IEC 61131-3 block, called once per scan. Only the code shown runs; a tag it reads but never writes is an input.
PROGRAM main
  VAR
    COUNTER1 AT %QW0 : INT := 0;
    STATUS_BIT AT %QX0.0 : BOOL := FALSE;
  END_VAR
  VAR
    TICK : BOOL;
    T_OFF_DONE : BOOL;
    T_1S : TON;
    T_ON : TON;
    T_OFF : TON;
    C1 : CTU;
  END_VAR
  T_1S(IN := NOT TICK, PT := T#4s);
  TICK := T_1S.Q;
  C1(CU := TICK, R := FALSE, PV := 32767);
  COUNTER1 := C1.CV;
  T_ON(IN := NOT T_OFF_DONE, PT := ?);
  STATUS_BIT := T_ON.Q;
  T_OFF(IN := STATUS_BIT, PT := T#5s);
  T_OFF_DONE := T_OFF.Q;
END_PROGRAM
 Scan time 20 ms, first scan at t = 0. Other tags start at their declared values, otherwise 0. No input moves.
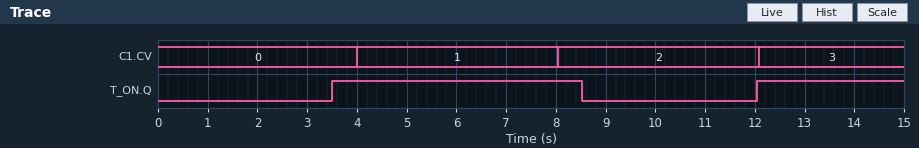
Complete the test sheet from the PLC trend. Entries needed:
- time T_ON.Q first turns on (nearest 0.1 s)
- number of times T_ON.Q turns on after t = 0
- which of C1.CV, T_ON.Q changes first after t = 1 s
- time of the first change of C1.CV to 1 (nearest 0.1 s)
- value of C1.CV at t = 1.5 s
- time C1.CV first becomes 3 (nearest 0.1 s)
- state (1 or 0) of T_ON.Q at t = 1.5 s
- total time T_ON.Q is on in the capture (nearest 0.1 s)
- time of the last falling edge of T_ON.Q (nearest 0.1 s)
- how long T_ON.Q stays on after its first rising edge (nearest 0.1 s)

3.5 s
2
T_ON.Q
4.0 s
0
12.1 s
0
8.0 s
8.5 s
5.0 s
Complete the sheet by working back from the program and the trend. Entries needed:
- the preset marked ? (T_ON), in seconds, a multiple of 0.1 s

3.5 s
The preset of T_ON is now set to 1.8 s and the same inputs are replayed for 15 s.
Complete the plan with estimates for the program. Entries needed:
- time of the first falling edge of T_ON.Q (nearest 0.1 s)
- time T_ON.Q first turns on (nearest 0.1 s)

6.8 s
1.8 s
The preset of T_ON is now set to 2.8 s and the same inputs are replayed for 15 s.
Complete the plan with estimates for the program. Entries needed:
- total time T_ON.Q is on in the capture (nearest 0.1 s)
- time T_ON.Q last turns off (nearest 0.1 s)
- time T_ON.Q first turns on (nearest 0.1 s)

9.4 s
7.8 s
2.8 s
